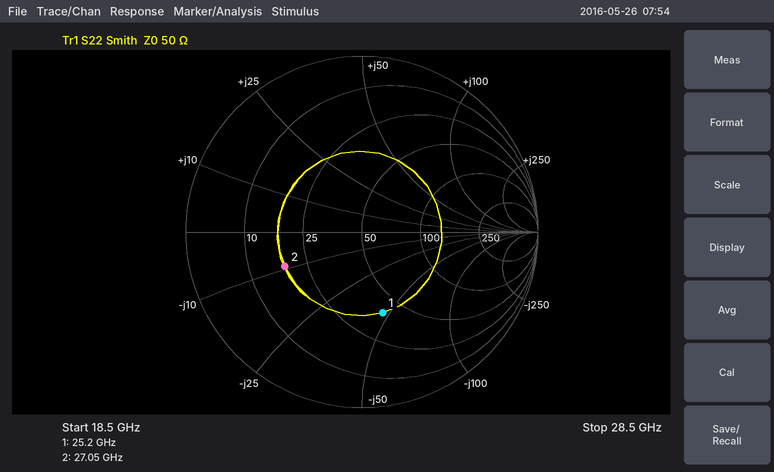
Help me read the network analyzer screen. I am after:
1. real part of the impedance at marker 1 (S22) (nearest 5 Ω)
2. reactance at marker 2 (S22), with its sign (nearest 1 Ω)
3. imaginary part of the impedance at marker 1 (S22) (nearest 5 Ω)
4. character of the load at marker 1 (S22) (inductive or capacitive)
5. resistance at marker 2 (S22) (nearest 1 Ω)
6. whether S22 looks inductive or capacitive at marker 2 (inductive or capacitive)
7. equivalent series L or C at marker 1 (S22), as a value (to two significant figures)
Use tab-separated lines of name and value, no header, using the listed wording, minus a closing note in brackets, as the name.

real part of the impedance at marker 1 (S22)	40 Ω
reactance at marker 2 (S22), with its sign	-9 Ω
imaginary part of the impedance at marker 1 (S22)	-45 Ω
character of the load at marker 1 (S22)	capacitive
resistance at marker 2 (S22)	18 Ω
whether S22 looks inductive or capacitive at marker 2	capacitive
equivalent series L or C at marker 1 (S22), as a value	140 fF
